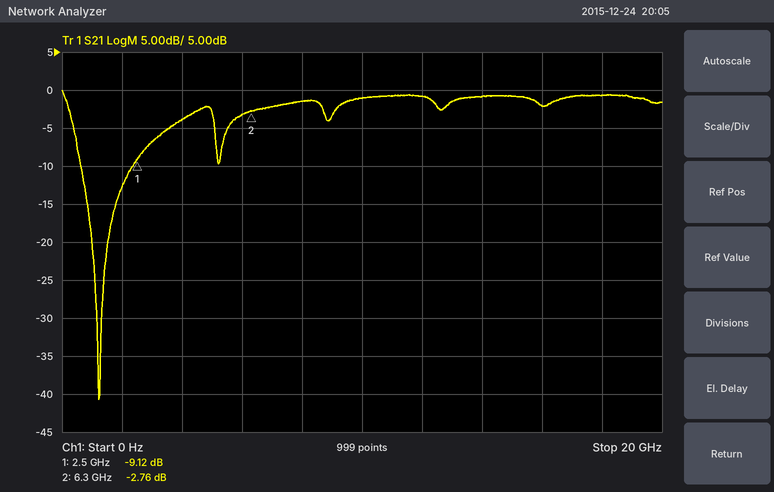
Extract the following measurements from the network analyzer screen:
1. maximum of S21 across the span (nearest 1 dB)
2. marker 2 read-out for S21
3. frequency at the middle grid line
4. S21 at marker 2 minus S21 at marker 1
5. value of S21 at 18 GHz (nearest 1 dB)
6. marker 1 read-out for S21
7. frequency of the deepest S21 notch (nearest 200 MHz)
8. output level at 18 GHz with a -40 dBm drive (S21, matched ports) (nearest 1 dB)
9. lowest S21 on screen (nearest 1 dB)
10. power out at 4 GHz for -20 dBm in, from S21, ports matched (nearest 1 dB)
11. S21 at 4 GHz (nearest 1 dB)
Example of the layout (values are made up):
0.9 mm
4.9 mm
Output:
0 dB
-2.76 dB
10 GHz
6.36 dB
-1 dB
-9.12 dB
1.2 GHz
-41 dBm
-41 dB
-24 dBm
-4 dB
